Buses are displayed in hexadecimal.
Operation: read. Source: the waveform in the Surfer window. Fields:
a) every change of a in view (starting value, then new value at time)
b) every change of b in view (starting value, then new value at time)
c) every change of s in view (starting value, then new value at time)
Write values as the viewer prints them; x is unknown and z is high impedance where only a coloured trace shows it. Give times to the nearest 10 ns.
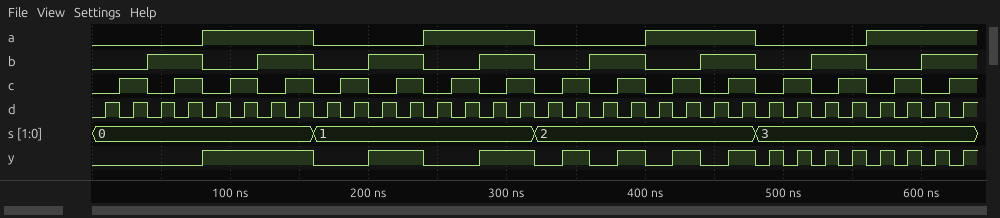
0, 1 at 80 ns, 0 at 160 ns, 1 at 240 ns, 0 at 320 ns, 1 at 400 ns, 0 at 480 ns, 1 at 560 ns
0, 1 at 40 ns, 0 at 80 ns, 1 at 120 ns, 0 at 160 ns, 1 at 200 ns, 0 at 240 ns, 1 at 280 ns, 0 at 320 ns, 1 at 360 ns, 0 at 400 ns, 1 at 440 ns, 0 at 480 ns, 1 at 520 ns, 0 at 560 ns, 1 at 600 ns
0, 1 at 160 ns, 2 at 320 ns, 3 at 480 ns
